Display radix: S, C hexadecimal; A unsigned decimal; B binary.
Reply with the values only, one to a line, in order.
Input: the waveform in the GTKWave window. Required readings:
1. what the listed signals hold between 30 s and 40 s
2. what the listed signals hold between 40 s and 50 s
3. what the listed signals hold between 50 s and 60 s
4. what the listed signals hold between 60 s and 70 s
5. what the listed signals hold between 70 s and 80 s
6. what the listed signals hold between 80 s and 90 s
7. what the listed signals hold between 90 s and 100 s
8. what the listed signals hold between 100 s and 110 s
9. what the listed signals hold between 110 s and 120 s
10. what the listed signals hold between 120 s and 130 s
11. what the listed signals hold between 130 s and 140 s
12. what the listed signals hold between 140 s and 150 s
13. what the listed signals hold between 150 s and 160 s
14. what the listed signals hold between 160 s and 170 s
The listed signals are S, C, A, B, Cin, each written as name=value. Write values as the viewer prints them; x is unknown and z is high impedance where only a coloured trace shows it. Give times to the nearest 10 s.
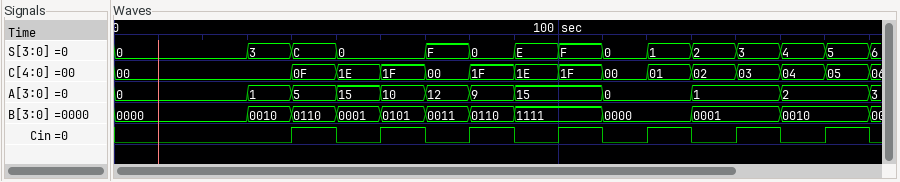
S=3, C=00, A=1, B=0010, Cin=0
S=C, C=0F, A=5, B=0110, Cin=1
S=0, C=1E, A=15, B=0001, Cin=0
S=0, C=1F, A=10, B=0101, Cin=1
S=F, C=00, A=12, B=0011, Cin=0
S=0, C=1F, A=9, B=0110, Cin=1
S=E, C=1E, A=15, B=1111, Cin=0
S=F, C=1F, A=15, B=1111, Cin=1
S=0, C=00, A=0, B=0000, Cin=0
S=1, C=01, A=0, B=0000, Cin=1
S=2, C=02, A=1, B=0001, Cin=0
S=3, C=03, A=1, B=0001, Cin=1
S=4, C=04, A=2, B=0010, Cin=0
S=5, C=05, A=2, B=0010, Cin=1
